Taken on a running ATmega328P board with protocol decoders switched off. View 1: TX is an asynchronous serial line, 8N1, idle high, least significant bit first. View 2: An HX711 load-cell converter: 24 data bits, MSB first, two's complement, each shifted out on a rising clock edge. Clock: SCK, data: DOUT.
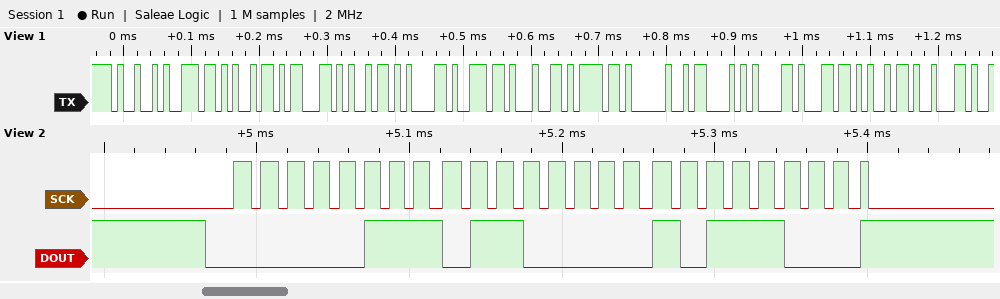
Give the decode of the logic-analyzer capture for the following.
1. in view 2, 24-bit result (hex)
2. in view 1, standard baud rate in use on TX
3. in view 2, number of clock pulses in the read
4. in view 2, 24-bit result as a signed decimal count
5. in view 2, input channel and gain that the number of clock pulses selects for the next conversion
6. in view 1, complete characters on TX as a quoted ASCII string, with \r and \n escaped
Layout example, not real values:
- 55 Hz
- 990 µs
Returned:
- 0x0760B8
- 115200 baud
- 25
- 483512
- channel A, gain 128
- "Iniciando Calib"
